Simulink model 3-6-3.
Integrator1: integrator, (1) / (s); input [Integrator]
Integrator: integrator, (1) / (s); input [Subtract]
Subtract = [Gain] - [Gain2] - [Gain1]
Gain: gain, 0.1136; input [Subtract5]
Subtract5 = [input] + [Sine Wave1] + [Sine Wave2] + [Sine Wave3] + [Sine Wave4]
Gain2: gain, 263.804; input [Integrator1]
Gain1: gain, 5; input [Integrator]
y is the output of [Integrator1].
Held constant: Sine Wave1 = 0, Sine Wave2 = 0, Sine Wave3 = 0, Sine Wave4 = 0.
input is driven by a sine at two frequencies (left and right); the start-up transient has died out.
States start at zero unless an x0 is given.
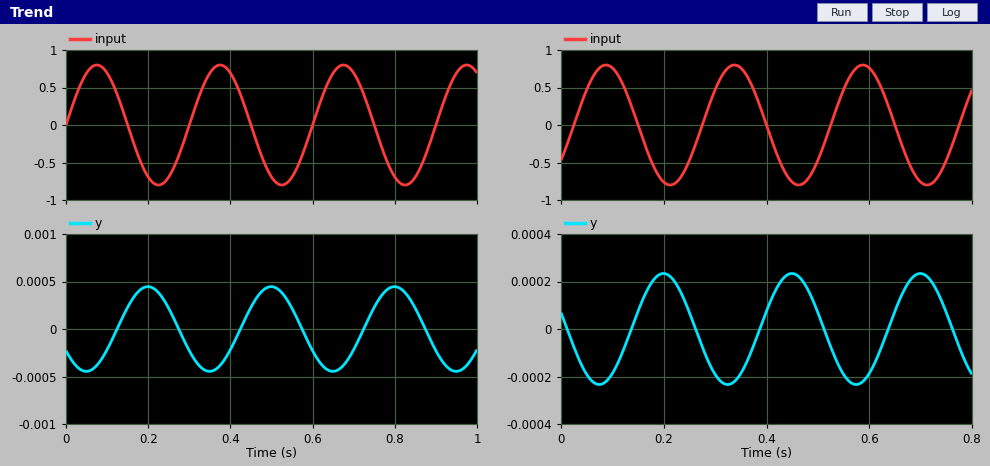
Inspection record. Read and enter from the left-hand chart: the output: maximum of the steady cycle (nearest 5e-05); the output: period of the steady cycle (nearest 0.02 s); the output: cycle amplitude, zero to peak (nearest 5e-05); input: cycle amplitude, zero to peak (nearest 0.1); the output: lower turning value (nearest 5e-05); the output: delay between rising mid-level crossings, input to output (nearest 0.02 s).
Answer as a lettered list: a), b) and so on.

a) 0.00045
b) 0.30 s
c) 0.00045
d) 0.8
e) -0.00045
f) 0.12 s
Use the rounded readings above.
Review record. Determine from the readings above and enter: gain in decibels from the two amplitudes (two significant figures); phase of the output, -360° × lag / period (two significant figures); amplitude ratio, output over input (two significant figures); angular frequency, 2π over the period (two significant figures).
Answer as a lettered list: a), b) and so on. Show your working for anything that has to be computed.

a) 20 log10(0.00045 / 0.8) = -65 dB
b) -360 × 0.12 / 0.3 = -140°
c) 0.00045 / 0.8 = 0.00056
d) 2π / 0.3 = 21 rad/s
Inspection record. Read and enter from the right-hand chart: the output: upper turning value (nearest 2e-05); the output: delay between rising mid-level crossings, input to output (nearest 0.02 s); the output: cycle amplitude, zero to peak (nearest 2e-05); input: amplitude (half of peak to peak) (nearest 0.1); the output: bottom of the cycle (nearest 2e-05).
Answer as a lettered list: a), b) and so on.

a) 0.00024
b) 0.12 s
c) 0.00024
d) 0.8
e) -0.00024
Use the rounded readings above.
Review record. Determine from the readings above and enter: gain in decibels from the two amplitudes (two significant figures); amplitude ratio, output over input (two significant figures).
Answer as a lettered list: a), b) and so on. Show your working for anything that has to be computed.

a) 20 log10(0.00024 / 0.8) = -70 dB
b) 0.00024 / 0.8 = 0.00030
